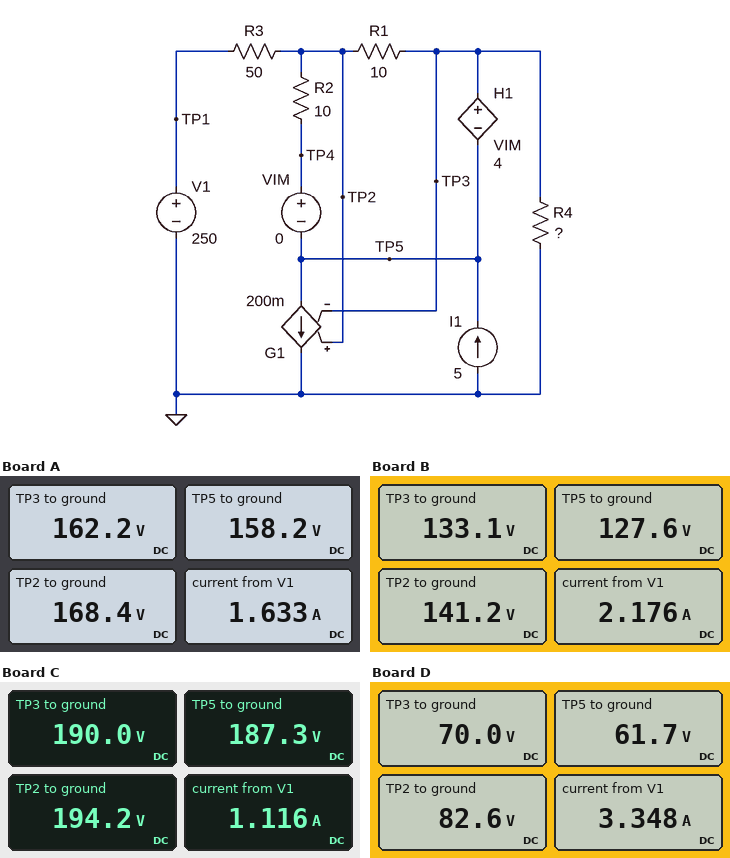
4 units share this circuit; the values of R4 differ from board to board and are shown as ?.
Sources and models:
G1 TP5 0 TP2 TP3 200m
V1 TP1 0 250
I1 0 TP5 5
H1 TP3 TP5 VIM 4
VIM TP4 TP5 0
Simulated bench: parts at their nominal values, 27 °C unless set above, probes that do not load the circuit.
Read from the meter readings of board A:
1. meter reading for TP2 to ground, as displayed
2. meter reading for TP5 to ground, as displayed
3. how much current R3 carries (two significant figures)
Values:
168.4 V
158.2 V
1.6 A
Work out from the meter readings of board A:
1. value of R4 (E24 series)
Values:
30 Ω
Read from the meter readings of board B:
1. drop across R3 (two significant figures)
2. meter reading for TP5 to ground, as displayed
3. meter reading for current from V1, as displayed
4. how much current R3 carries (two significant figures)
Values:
110 V
127.6 V
2.176 A
2.2 A
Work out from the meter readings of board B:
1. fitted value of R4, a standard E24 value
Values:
24 Ω
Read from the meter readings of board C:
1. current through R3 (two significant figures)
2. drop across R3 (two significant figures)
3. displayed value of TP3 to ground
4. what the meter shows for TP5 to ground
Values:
1.1 A
56 V
190.0 V
187.3 V
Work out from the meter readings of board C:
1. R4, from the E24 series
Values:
36 Ω
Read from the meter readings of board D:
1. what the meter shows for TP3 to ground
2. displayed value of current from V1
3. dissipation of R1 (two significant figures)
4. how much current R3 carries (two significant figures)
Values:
70.0 V
3.348 A
16 W
3.3 A
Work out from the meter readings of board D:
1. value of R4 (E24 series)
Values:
12 Ω
